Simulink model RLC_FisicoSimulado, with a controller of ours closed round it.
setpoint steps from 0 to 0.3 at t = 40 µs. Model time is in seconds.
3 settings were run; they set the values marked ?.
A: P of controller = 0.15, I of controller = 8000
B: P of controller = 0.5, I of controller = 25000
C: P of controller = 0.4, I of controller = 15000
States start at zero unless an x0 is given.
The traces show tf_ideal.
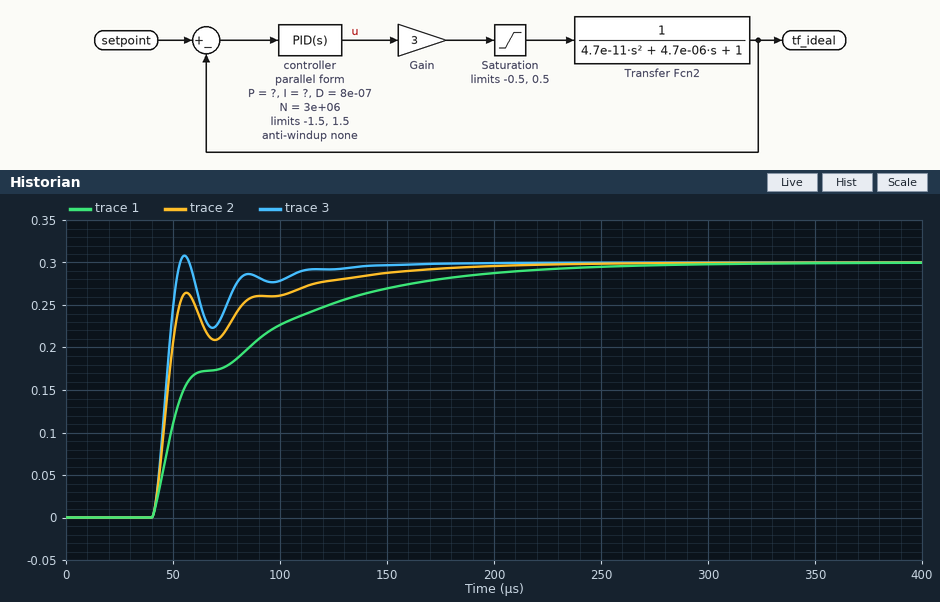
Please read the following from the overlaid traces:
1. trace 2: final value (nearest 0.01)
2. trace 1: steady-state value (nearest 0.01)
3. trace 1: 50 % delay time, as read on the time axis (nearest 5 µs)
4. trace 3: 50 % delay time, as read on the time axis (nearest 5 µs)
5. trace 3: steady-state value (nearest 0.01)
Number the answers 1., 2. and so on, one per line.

1. 0.30
2. 0.30
3. 55 µs
4. 45 µs
5. 0.30
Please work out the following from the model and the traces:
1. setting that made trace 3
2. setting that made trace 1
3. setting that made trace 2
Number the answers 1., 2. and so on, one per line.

1. B
2. A
3. C
